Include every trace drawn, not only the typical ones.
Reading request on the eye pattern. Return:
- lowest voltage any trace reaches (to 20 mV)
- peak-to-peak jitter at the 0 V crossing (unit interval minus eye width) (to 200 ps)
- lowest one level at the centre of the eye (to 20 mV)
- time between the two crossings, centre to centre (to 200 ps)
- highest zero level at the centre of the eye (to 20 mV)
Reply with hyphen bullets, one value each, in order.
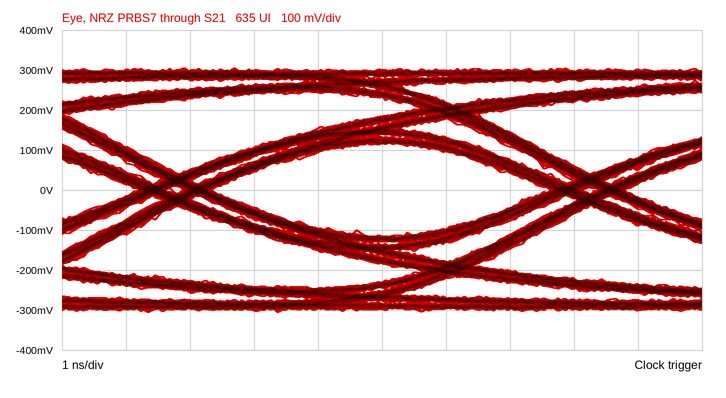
- -300 mV
- 1.2 ns
- 120 mV
- 6.4 ns
- -120 mV
